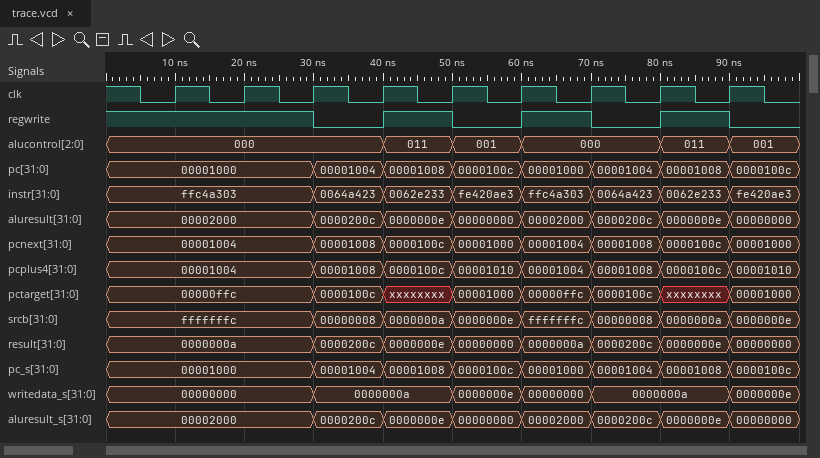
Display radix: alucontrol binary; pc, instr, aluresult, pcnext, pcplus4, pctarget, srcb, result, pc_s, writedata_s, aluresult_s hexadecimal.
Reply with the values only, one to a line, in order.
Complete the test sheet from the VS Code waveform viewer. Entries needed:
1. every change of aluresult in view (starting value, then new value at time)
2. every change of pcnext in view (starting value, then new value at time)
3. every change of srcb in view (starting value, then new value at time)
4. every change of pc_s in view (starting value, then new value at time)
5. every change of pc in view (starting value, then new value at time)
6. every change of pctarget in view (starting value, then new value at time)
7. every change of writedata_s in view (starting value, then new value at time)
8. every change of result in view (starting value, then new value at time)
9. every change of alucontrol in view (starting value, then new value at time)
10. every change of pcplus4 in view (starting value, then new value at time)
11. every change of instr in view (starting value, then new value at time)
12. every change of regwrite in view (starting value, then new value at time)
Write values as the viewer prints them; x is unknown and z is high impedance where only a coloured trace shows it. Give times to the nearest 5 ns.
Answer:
00002000, 0000200c at 30 ns, 0000000e at 40 ns, 00000000 at 50 ns, 00002000 at 60 ns, 0000200c at 70 ns, 0000000e at 80 ns, 00000000 at 90 ns
00001004, 00001008 at 30 ns, 0000100c at 40 ns, 00001000 at 50 ns, 00001004 at 60 ns, 00001008 at 70 ns, 0000100c at 80 ns, 00001000 at 90 ns
fffffffc, 00000008 at 30 ns, 0000000a at 40 ns, 0000000e at 50 ns, fffffffc at 60 ns, 00000008 at 70 ns, 0000000a at 80 ns, 0000000e at 90 ns
00001000, 00001004 at 30 ns, 00001008 at 40 ns, 0000100c at 50 ns, 00001000 at 60 ns, 00001004 at 70 ns, 00001008 at 80 ns, 0000100c at 90 ns
00001000, 00001004 at 30 ns, 00001008 at 40 ns, 0000100c at 50 ns, 00001000 at 60 ns, 00001004 at 70 ns, 00001008 at 80 ns, 0000100c at 90 ns
00000ffc, 0000100c at 30 ns, xxxxxxxx at 40 ns, 00001000 at 50 ns, 00000ffc at 60 ns, 0000100c at 70 ns, xxxxxxxx at 80 ns, 00001000 at 90 ns
00000000, 0000000a at 30 ns, 0000000e at 50 ns, 00000000 at 60 ns, 0000000a at 70 ns, 0000000e at 90 ns
0000000a, 0000200c at 30 ns, 0000000e at 40 ns, 00000000 at 50 ns, 0000000a at 60 ns, 0000200c at 70 ns, 0000000e at 80 ns, 00000000 at 90 ns
000, 011 at 40 ns, 001 at 50 ns, 000 at 60 ns, 011 at 80 ns, 001 at 90 ns
00001004, 00001008 at 30 ns, 0000100c at 40 ns, 00001010 at 50 ns, 00001004 at 60 ns, 00001008 at 70 ns, 0000100c at 80 ns, 00001010 at 90 ns
ffc4a303, 0064a423 at 30 ns, 0062e233 at 40 ns, fe420ae3 at 50 ns, ffc4a303 at 60 ns, 0064a423 at 70 ns, 0062e233 at 80 ns, fe420ae3 at 90 ns
1, 0 at 30 ns, 1 at 40 ns, 0 at 50 ns, 1 at 60 ns, 0 at 70 ns, 1 at 80 ns, 0 at 90 ns
